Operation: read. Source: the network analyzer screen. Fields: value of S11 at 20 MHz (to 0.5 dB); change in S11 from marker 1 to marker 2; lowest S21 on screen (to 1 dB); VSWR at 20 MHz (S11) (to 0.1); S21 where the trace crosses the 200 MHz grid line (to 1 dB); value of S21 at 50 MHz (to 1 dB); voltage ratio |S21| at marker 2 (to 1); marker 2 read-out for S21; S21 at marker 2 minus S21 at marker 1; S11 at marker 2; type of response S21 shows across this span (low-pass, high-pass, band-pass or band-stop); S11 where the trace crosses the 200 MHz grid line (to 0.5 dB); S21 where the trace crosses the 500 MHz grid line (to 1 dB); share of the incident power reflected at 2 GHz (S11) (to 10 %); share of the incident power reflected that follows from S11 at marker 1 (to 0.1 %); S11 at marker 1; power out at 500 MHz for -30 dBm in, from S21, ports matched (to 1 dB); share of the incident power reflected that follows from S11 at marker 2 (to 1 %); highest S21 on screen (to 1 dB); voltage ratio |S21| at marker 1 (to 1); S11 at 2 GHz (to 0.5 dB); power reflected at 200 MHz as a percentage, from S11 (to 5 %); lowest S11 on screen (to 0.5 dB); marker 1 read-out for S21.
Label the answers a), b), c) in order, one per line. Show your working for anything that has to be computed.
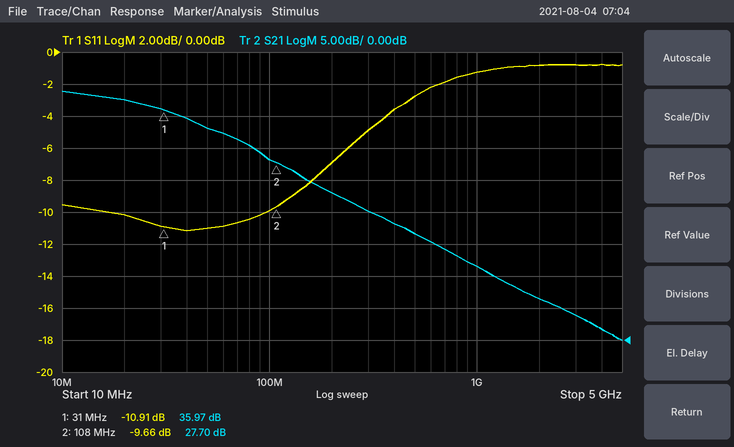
a) -10.0 dB
b) -9.66 − (-10.91) = 1.25 dB
c) 0 dB
d) |Γ| = 10^(-10/20) = 0.3162; VSWR = (1 + 0.3162)/(1 − 0.3162) ≈ 1.9
e) 23 dB
f) 33 dB
g) 10^(27.7/20) ≈ 24
h) 27.70 dB
i) 27.7 − (35.97) = -8.27 dB
j) -9.66 dB
k) low-pass
l) -7.0 dB
m) 17 dB
n) 10^(-1/10) ≈ 79.4 %, so 80 % to the nearest 10 %
o) 10^(-10.91/10) ≈ 8.1 %
p) -10.91 dB
q) -30 dBm + (17 dB) = -13 dBm
r) 10^(-9.66/10) ≈ 11 %
s) 39 dB
t) 10^(35.97/20) ≈ 63
u) -1.0 dB
v) 10^(-7/10) ≈ 20 %
w) -11.0 dB
x) 35.97 dB
